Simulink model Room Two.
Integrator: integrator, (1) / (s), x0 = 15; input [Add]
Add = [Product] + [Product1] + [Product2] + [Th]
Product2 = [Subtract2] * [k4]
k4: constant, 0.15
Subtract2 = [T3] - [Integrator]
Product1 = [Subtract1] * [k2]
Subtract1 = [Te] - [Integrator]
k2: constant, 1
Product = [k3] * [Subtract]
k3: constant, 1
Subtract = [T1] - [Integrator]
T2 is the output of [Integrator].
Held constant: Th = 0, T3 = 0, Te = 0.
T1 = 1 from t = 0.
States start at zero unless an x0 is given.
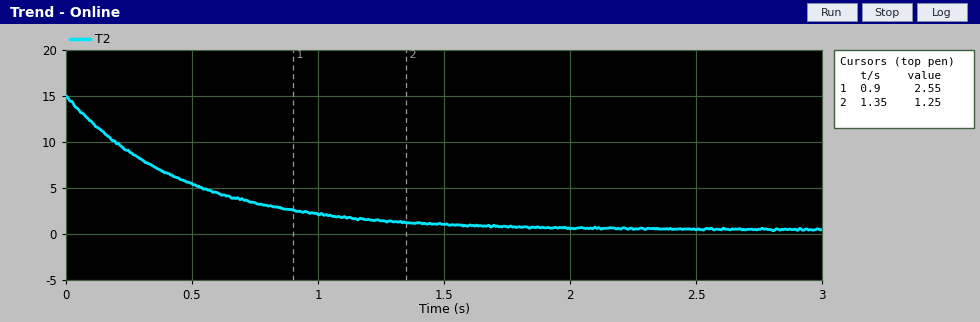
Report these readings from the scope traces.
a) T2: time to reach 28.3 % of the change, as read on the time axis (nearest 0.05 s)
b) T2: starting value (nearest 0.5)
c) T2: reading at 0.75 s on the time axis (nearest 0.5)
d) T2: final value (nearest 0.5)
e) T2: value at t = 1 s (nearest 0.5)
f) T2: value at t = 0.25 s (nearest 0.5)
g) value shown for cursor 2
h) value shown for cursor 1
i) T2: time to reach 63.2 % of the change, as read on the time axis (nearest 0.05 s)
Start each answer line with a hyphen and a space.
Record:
- 0.15 s
- 15.0
- 3.5
- 0.5
- 2.0
- 9.0
- 1.25
- 2.55
- 0.45 s
